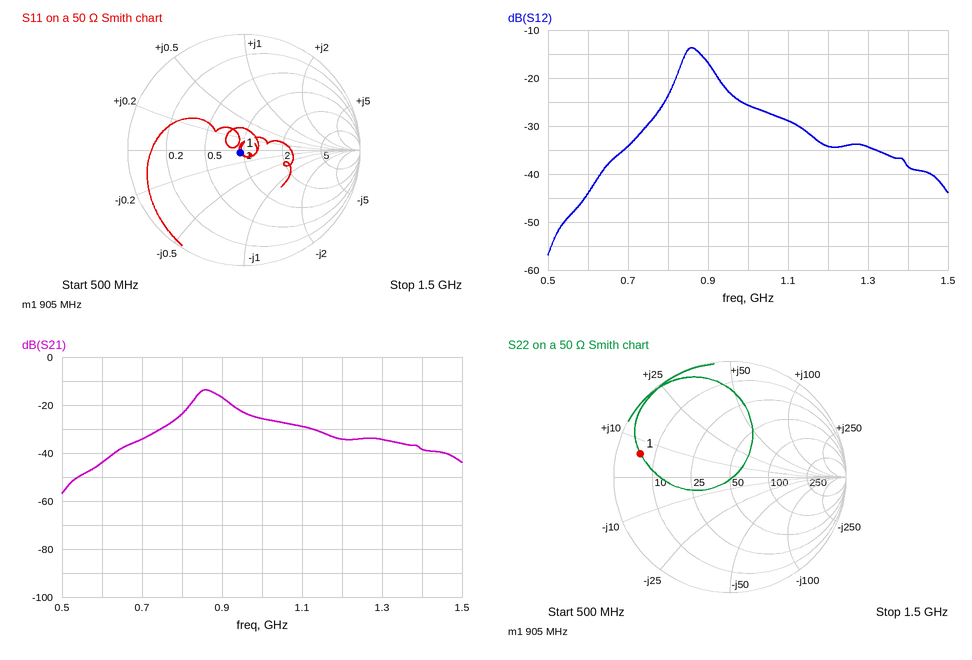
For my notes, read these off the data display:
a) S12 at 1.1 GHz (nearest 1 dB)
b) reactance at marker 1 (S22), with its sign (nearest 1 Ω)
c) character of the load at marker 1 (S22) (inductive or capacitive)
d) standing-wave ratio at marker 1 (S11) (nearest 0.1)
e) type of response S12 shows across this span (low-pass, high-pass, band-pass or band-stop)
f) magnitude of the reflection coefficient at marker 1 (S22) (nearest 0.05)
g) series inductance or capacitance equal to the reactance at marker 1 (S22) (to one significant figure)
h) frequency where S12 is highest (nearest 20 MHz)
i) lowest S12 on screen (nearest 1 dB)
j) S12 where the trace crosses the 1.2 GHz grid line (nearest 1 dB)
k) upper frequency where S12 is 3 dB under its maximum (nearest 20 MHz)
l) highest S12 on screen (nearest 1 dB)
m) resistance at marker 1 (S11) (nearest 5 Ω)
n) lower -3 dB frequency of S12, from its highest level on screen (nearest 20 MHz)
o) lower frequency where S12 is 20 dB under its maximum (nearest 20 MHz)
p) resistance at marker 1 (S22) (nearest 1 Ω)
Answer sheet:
-29 dB
+6 Ω
inductive
1.1
band-pass
0.80
1 nH
860 MHz
-57 dB
-34 dB
900 MHz
-14 dB
45 Ω
840 MHz
700 MHz
6 Ω
